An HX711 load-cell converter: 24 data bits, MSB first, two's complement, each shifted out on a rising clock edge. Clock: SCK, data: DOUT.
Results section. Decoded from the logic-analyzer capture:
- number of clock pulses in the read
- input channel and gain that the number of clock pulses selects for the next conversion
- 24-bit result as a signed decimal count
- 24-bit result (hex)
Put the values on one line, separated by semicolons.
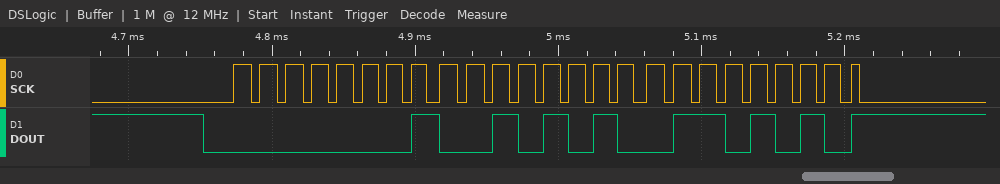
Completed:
25; channel A, gain 128; 76394; 0x012A6A
